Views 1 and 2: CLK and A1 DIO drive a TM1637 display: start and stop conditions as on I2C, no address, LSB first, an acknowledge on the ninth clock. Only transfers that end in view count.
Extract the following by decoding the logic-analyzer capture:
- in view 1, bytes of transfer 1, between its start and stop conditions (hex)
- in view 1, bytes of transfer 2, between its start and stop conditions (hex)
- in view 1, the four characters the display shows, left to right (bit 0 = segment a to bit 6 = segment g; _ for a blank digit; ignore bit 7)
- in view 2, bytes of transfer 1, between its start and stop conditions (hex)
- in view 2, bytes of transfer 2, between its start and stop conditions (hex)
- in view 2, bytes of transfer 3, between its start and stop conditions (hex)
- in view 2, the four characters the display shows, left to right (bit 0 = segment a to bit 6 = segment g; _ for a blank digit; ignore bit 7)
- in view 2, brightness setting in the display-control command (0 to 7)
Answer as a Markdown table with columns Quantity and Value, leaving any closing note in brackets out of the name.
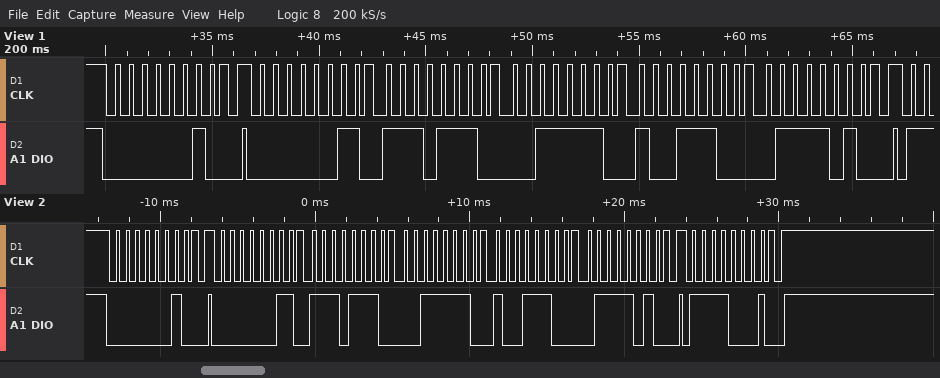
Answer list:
| Quantity | Value |
|---|---|
| in view 1, bytes of transfer 1, between its start and stop conditions | 40 |
| in view 1, bytes of transfer 2, between its start and stop conditions | C0 77 7C 39 5E |
| in view 1, the four characters the display shows, left to right | AbCd |
| in view 2, bytes of transfer 1, between its start and stop conditions | 40 |
| in view 2, bytes of transfer 2, between its start and stop conditions | C0 77 7C 39 5E |
| in view 2, bytes of transfer 3, between its start and stop conditions | 8F |
| in view 2, the four characters the display shows, left to right | AbCd |
| in view 2, brightness setting in the display-control command | 7 |
